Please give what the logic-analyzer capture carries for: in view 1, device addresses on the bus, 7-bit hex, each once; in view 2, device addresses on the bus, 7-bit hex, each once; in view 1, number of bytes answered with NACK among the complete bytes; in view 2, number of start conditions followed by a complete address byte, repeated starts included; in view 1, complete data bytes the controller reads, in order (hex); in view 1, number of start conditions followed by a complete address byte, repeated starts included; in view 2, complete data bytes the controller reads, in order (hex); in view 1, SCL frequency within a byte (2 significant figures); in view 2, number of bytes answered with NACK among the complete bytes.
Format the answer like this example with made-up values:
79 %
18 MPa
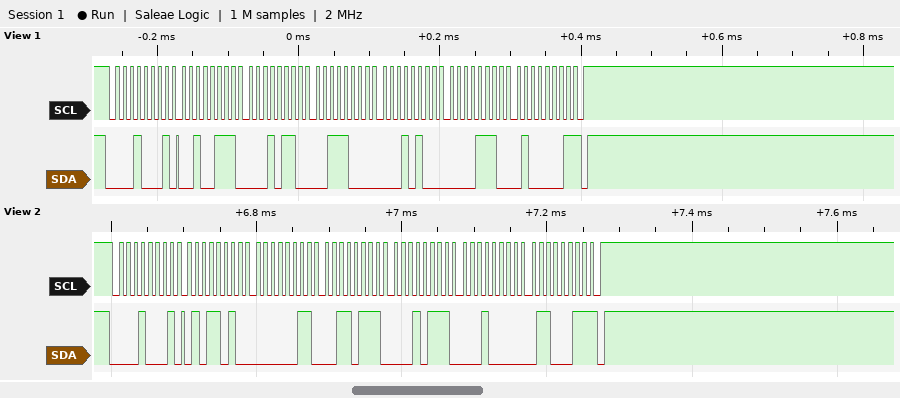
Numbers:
0x08
0x08
1
1
27 16 38 14 0E 41
1
5A 03 37 17 10 63
100 kHz
1
